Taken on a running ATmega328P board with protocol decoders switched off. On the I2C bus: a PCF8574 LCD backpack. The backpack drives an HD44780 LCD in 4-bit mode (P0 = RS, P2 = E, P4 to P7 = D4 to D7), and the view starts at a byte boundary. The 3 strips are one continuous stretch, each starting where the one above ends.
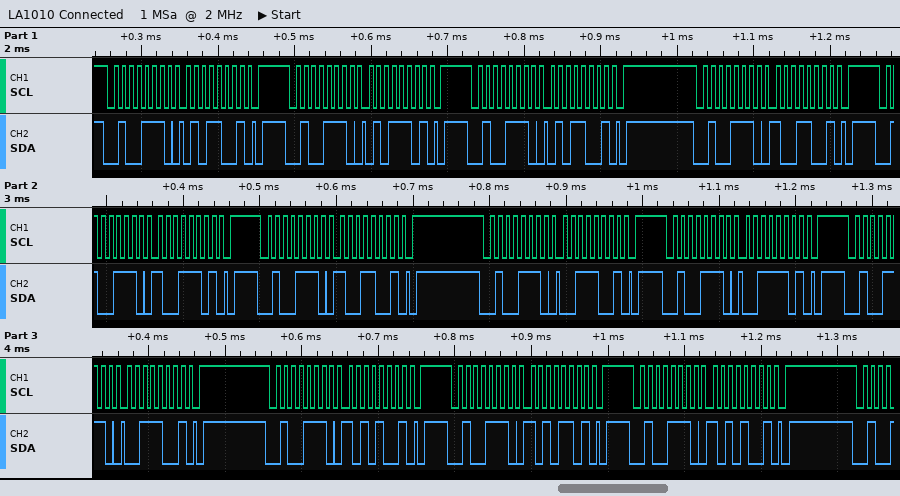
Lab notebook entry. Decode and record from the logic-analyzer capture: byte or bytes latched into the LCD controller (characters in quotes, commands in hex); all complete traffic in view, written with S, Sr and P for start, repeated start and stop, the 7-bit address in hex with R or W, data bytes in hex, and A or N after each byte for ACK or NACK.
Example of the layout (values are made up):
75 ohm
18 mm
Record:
'Y' ':'
S 27W A 59 A P S 27W A 5D A P S 27W A 59 A P S 27W A 99 A P S 27W A 9D A P S 27W A 99 A P S 27W A 39 A P S 27W A 3D A P S 27W A 39 A P S 27W A A9 A P S 27W A AD A P S 27W A A9 A P
